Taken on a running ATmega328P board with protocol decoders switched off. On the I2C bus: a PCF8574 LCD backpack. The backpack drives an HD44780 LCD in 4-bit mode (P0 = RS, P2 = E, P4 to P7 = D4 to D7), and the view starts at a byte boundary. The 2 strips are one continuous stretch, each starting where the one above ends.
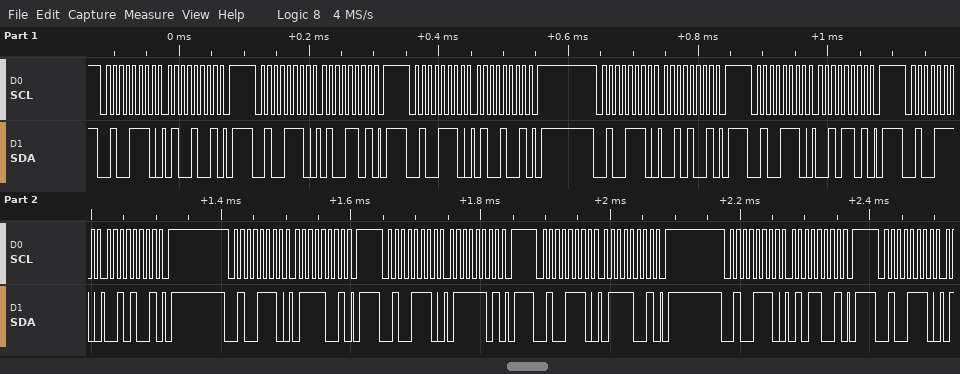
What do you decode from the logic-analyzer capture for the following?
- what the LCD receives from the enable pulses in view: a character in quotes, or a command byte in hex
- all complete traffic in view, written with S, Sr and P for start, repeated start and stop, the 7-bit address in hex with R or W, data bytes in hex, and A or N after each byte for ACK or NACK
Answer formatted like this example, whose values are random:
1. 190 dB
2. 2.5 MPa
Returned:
1. 'B'
2. S 27W A 49 A P S 27W A 4D A P S 27W A 49 A P S 27W A 29 A P S 27W A 2D A P S 27W A 29 A P S 27W A 79 A P S 27W A 7D A P S 27W A 79 A P S 27W A 59 A P S 27W A
